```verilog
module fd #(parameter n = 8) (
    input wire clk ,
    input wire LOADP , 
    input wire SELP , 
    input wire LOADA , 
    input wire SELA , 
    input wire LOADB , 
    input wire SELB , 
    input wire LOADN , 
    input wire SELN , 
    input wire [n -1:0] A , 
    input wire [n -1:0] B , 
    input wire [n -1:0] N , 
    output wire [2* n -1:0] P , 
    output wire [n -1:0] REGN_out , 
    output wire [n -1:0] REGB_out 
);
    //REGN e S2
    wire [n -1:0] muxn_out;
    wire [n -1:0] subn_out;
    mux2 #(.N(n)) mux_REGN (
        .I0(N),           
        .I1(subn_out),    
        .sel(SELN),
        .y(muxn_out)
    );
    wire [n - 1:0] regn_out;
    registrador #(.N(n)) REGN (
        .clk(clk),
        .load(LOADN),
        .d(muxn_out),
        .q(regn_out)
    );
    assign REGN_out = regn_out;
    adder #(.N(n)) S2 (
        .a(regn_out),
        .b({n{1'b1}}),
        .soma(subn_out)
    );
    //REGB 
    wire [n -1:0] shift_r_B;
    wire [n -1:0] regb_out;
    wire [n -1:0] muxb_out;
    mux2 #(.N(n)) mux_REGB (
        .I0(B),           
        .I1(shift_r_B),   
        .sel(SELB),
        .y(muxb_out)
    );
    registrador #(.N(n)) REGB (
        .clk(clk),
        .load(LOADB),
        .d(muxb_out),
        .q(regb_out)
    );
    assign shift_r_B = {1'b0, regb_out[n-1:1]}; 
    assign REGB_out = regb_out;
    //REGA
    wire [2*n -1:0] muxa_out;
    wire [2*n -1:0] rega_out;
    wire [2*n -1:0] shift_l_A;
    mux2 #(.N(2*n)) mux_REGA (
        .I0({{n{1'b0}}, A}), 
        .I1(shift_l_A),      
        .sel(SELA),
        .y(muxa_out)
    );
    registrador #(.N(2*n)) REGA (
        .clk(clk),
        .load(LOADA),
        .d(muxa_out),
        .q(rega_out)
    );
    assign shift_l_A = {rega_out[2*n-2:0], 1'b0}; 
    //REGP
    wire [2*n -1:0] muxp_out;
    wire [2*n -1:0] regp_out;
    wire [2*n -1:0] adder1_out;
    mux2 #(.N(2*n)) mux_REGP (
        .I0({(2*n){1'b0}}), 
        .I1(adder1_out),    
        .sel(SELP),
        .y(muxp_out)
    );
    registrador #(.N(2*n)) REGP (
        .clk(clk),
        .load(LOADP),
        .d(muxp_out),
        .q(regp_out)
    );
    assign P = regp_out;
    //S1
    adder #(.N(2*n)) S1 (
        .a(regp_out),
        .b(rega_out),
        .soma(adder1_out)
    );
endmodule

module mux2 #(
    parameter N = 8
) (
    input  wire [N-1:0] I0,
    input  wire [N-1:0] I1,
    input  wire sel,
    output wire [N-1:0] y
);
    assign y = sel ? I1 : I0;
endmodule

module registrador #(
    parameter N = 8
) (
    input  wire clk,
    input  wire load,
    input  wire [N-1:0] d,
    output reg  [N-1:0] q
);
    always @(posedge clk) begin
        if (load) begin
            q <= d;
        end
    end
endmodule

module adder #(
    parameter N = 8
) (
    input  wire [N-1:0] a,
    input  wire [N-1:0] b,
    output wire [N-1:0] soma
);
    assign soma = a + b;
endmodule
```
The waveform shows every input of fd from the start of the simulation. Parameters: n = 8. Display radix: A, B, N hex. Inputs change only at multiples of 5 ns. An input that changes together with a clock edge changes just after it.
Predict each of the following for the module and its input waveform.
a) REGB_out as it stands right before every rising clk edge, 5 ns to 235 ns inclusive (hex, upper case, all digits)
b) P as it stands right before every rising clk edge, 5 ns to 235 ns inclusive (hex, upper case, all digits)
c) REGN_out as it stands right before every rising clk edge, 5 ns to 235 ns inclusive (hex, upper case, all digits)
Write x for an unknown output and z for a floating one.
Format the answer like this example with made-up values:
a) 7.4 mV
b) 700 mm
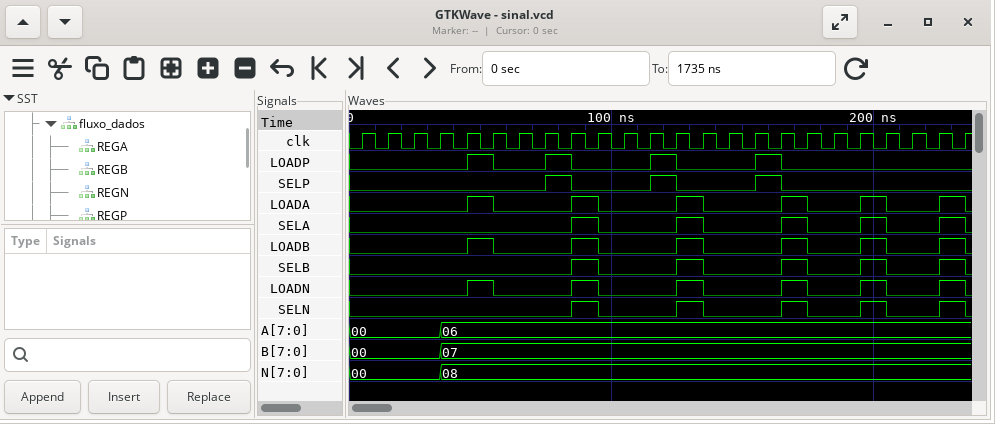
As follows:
a) x, x, x, x, x, x, 07, 07, 07, 07, 03, 03, 03, 03, 01, 01, 01, 01, 00, 00, 00, 00, 00, 00
b) x, x, x, x, x, x, 0000, 0000, 0000, 0006, 0006, 0006, 0006, 0012, 0012, 0012, 0012, 002A, 002A, 002A, 002A, 002A, 002A, 002A
c) x, x, x, x, x, x, 08, 08, 08, 08, 07, 07, 07, 07, 06, 06, 06, 06, 05, 05, 05, 04, 04, 04
